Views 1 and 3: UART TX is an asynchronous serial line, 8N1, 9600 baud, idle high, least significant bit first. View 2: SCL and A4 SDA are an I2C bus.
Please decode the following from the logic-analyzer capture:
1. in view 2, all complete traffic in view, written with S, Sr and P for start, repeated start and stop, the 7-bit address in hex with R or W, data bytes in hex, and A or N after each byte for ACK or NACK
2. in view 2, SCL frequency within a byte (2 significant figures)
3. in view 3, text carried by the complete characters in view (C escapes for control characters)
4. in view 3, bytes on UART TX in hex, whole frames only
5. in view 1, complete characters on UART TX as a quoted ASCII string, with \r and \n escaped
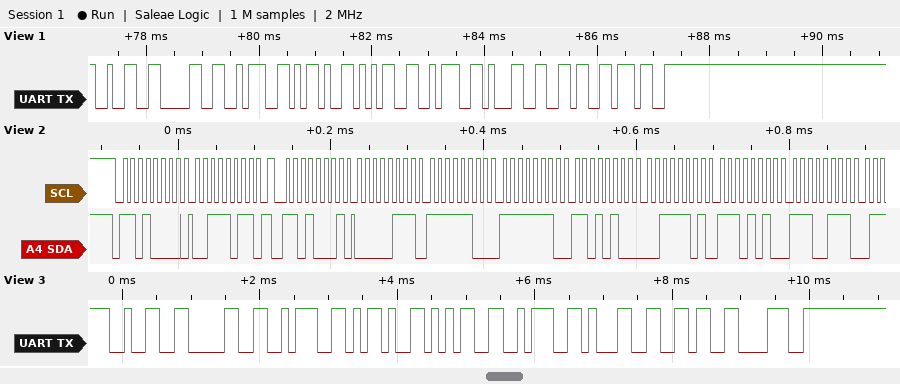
S 68W A 3B A Sr 68R A 07 A FC A FE A D4 A 3D A EA A E7 A
100 kHz
"20:-5:168"
32 30 3A 2D 35 3A 31 36 38
"20:-5:167"
